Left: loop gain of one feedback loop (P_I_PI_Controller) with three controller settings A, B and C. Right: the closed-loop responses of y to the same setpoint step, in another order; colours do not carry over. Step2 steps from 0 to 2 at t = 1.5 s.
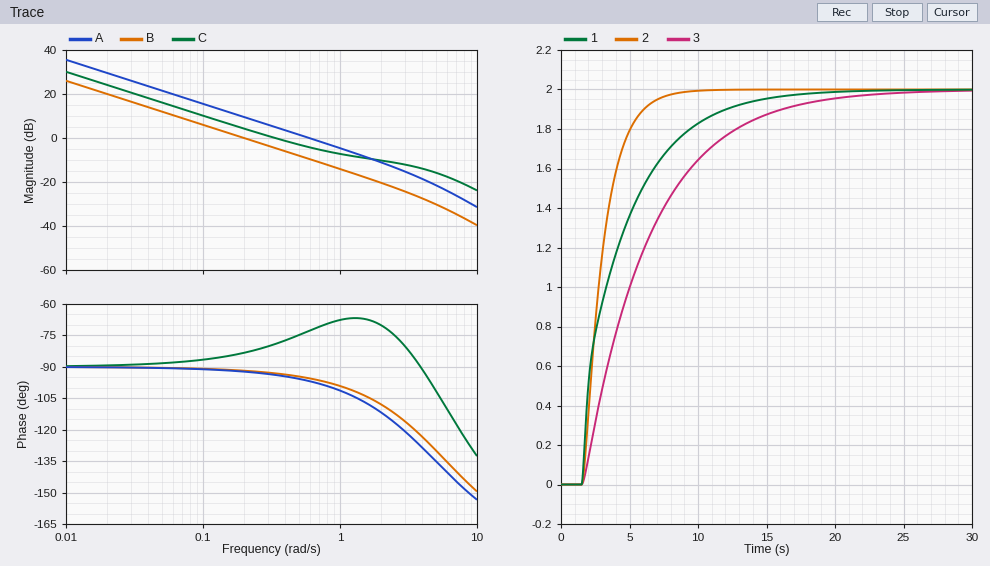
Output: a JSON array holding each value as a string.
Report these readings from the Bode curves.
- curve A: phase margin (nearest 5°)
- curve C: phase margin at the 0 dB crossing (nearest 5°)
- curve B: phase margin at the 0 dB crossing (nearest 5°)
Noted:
["85°", "100°", "90°"]
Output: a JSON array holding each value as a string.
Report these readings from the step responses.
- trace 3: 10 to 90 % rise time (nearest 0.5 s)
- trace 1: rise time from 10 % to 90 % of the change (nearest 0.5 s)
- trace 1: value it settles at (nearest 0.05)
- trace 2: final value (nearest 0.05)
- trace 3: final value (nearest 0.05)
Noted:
["10.5 s", "7.5 s", "2.00", "2.00", "2.00"]
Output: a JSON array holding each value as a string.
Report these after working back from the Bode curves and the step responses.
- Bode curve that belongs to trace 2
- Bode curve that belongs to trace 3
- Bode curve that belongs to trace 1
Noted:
["A", "B", "C"]
